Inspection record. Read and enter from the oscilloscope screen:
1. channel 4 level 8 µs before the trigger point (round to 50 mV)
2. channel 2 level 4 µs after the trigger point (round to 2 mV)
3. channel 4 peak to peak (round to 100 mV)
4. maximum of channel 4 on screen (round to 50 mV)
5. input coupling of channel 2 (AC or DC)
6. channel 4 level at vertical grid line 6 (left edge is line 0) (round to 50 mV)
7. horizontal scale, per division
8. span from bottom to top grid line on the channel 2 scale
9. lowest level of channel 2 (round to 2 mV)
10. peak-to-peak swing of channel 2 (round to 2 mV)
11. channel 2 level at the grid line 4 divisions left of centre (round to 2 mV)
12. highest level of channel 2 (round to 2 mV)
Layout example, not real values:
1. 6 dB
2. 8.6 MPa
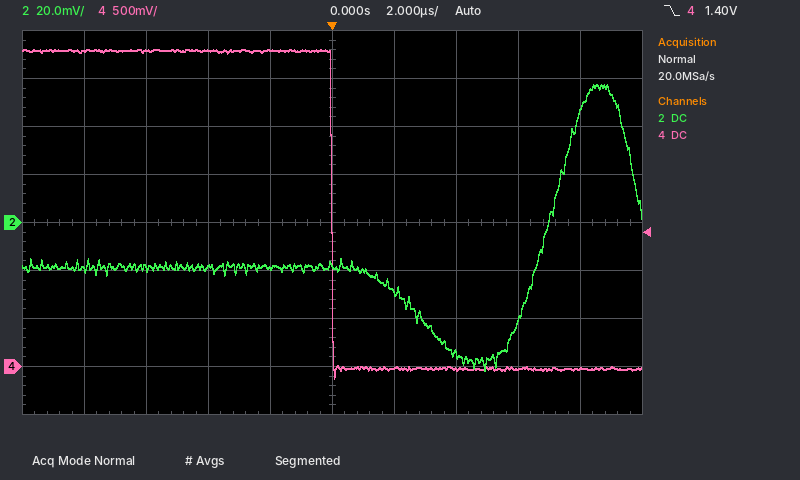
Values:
1. 3.30 V
2. -54 mV
3. 3.40 V
4. 3.30 V
5. DC
6. 0 mV
7. 2 µs
8. 160 mV
9. -62 mV
10. 120 mV
11. -20 mV
12. 58 mV
